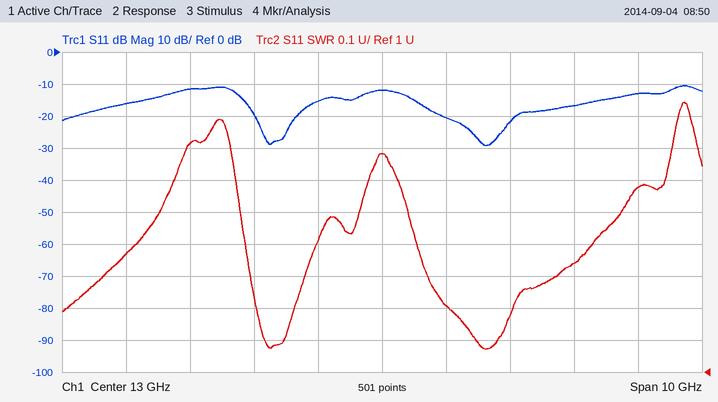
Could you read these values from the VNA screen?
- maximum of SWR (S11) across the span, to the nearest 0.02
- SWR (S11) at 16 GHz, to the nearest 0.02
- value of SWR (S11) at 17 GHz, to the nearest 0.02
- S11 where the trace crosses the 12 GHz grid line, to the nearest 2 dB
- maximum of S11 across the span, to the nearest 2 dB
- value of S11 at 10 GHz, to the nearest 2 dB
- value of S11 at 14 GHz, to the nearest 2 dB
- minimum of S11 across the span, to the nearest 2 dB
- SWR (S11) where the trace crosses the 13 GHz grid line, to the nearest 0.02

1.84
1.34
1.58
-16 dB
-10 dB
-12 dB
-20 dB
-30 dB
1.68
